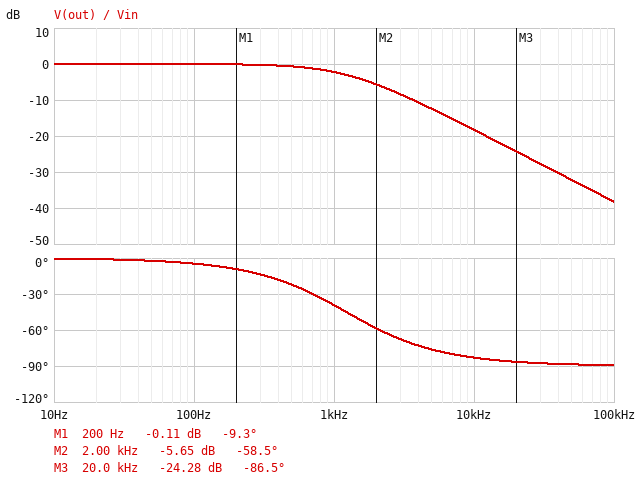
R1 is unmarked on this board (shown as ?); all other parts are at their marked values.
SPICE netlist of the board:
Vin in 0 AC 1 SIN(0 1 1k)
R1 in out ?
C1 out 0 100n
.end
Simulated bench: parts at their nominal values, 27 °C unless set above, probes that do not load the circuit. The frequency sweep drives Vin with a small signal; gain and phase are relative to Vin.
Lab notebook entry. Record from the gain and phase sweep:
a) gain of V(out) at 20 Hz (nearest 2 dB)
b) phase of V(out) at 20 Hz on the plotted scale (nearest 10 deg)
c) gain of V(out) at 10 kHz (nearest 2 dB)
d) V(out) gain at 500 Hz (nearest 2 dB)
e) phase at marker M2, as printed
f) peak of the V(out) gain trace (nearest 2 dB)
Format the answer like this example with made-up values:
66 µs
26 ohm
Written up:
0 dB
0 deg
-18 dB
0 dB
-58.5 deg
0 dB
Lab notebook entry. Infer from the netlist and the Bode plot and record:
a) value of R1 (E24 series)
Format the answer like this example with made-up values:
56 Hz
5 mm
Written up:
1.3 kΩ
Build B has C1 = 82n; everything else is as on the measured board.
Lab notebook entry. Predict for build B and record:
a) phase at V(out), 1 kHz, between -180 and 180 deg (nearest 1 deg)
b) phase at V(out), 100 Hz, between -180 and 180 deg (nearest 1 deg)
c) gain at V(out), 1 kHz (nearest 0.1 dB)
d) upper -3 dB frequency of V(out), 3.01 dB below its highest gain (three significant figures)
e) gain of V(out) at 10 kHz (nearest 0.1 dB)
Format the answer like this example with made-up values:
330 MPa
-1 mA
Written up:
-34 deg
-4 deg
-1.6 dB
1.49 kHz
-16.6 dB
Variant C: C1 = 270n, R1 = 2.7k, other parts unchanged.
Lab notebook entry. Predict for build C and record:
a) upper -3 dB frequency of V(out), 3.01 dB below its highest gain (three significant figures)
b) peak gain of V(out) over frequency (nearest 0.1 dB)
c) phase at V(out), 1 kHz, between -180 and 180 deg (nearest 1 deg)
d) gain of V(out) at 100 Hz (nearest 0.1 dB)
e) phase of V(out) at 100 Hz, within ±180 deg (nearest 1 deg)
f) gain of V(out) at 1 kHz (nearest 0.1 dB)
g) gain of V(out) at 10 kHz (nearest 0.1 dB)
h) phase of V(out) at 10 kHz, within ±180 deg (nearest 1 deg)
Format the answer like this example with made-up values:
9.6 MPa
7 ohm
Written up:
218 Hz
0 dB
-78 deg
-0.8 dB
-25 deg
-13.4 dB
-33.2 dB
-89 deg
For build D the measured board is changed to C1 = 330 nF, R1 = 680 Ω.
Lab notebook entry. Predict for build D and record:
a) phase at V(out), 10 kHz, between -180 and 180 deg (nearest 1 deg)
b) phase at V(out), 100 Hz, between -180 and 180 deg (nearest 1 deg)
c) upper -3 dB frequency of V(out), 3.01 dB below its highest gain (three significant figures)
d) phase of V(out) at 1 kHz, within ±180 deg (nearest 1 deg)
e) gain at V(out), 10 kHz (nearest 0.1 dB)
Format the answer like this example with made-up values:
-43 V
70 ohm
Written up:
-86 deg
-8 deg
709 Hz
-55 deg
-23.0 dB
